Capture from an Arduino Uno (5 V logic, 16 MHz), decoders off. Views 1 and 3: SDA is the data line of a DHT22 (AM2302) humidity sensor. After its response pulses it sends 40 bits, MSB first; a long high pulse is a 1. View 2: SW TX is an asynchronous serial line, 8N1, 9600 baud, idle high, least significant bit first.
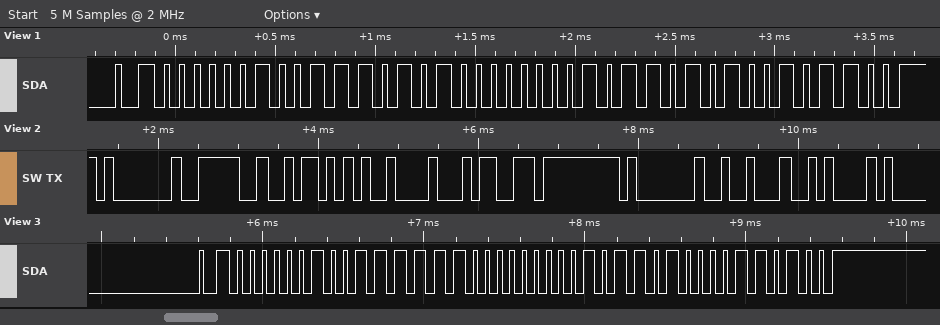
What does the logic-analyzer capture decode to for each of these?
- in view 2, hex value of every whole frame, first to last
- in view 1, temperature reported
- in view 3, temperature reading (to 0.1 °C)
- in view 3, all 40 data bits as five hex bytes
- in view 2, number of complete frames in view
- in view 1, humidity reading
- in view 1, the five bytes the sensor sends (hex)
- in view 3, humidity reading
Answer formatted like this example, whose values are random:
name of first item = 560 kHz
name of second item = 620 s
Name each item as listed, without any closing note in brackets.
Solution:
in view 2, hex value of every whole frame, first to last = 0x01 0x3E 0x5A 0x09 0x34 0xFF 0x01 0x12 0x0A
in view 1, temperature reported = 18.1 °C
in view 3, temperature reading = 18.0 °C
in view 3, all 40 data bits as five hex bytes = 02 7E 00 B4 34
in view 2, number of complete frames in view = 9
in view 1, humidity reading = 62.9 %
in view 1, the five bytes the sensor sends = 02 75 00 B5 2C
in view 3, humidity reading = 63.8 %
